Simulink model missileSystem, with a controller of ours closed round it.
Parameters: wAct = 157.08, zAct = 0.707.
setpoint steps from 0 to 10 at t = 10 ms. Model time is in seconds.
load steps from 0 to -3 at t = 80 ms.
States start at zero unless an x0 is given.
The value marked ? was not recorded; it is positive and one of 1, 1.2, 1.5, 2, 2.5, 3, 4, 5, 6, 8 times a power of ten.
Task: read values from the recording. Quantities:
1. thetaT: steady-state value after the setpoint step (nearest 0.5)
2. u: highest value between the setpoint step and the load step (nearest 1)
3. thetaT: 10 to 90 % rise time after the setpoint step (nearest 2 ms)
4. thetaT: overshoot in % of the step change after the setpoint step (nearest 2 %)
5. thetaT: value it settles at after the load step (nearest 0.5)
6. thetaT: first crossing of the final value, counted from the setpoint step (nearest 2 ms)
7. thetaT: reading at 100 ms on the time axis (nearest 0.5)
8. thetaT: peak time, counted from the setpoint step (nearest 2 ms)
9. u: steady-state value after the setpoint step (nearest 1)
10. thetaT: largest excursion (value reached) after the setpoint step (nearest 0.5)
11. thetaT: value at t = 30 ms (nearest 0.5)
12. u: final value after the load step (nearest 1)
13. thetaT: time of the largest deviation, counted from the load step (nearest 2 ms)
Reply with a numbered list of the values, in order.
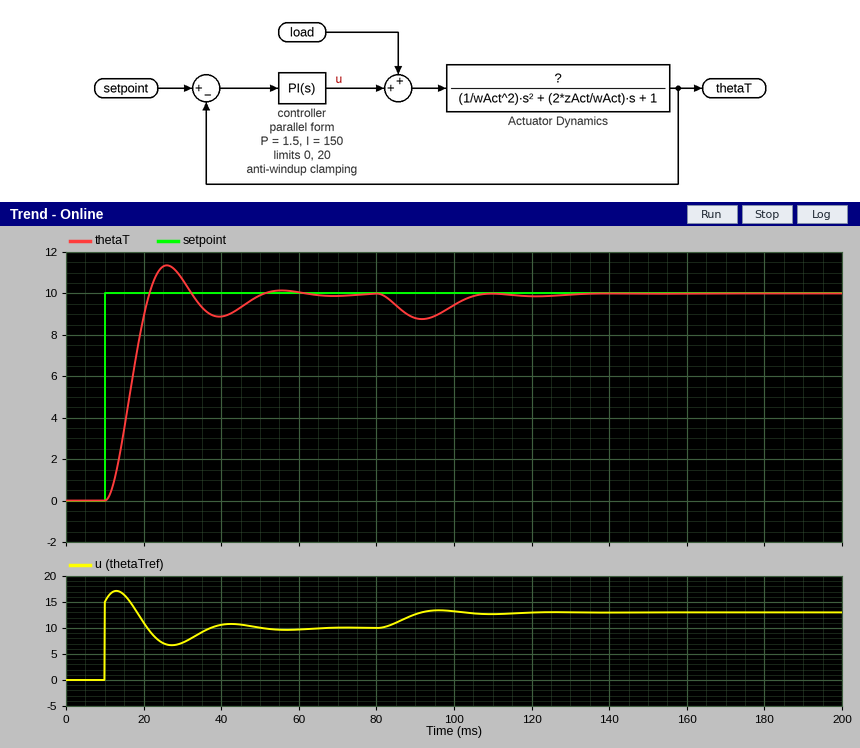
1. 10.0
2. 17
3. 8 ms
4. 14 %
5. 10.0
6. 12 ms
7. 9.5
8. 16 ms
9. 10
10. 11.5
11. 10.5
12. 13
13. 12 ms
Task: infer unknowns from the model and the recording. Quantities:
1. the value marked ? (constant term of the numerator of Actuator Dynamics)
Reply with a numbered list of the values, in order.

1. 1
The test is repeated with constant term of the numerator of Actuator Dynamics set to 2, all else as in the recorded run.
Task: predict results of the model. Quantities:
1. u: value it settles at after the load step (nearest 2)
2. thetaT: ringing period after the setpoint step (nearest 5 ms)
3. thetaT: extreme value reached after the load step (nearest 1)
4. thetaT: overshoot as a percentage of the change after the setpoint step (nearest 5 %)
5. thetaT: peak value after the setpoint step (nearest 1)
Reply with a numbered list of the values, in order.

1. 8
2. 20 ms
3. 8
4. 35 %
5. 13
